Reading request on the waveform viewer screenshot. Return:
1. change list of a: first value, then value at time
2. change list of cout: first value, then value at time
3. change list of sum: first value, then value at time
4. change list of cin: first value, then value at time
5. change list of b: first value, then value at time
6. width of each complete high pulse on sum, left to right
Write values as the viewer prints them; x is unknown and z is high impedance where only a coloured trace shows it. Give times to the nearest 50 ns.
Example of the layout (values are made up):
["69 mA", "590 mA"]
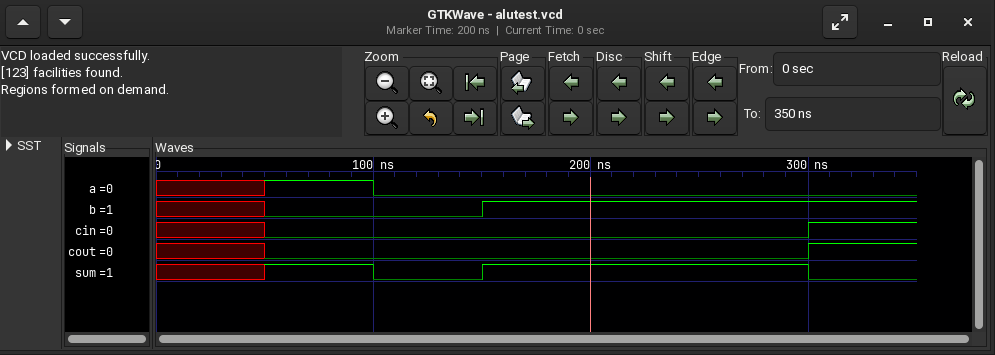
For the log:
["x, 1 at 50 ns, 0 at 100 ns", "x, 0 at 50 ns, 1 at 300 ns", "x, 1 at 50 ns, 0 at 100 ns, 1 at 150 ns, 0 at 300 ns", "x, 0 at 50 ns, 1 at 300 ns", "x, 0 at 50 ns, 1 at 150 ns", "150 ns"]
